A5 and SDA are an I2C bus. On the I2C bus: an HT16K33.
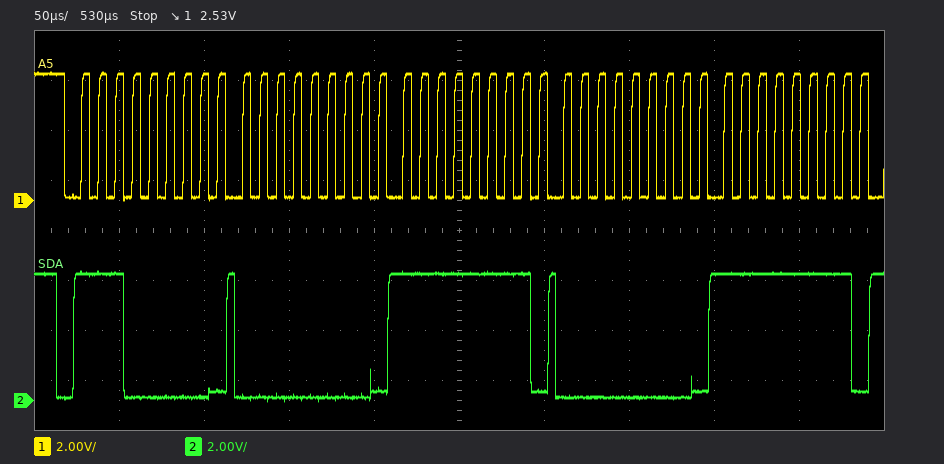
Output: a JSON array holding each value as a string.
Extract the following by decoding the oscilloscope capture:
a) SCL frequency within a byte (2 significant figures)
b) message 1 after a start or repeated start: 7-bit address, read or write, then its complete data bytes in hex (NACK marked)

["100 kHz", "0x70 write: 00 FF 00 FF"]
